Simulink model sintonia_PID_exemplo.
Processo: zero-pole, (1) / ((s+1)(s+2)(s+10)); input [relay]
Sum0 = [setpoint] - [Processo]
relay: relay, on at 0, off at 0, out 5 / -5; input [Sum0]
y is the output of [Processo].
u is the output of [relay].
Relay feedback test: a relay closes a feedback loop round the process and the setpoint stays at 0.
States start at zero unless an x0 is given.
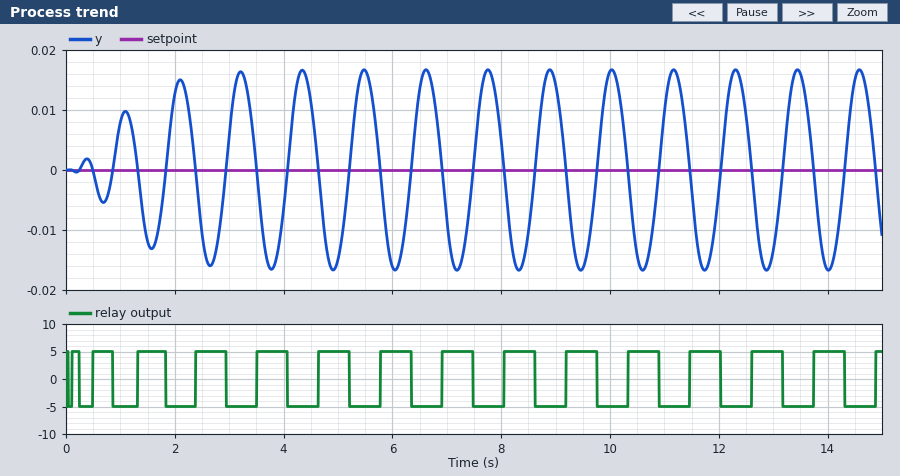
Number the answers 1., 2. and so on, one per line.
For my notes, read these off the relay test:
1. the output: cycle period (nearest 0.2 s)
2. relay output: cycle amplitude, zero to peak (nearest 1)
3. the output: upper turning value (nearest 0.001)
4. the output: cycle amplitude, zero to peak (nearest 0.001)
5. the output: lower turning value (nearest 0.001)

1. 1.2 s
2. 5
3. 0.017
4. 0.017
5. -0.017
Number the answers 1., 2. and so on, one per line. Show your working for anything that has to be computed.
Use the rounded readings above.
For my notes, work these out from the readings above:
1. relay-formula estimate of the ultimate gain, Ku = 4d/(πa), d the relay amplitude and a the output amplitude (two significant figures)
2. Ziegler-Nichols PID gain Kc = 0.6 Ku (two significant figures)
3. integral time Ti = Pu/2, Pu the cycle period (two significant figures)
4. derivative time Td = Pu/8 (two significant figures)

1. 4 × 5 / (π × 0.017) = 370
2. 0.6 × 370 = 220
3. 1.2 / 2 = 0.60 s
4. 1.2 / 8 = 0.15 s
